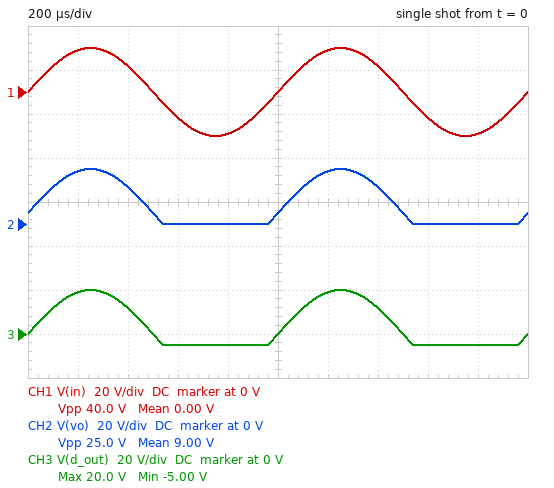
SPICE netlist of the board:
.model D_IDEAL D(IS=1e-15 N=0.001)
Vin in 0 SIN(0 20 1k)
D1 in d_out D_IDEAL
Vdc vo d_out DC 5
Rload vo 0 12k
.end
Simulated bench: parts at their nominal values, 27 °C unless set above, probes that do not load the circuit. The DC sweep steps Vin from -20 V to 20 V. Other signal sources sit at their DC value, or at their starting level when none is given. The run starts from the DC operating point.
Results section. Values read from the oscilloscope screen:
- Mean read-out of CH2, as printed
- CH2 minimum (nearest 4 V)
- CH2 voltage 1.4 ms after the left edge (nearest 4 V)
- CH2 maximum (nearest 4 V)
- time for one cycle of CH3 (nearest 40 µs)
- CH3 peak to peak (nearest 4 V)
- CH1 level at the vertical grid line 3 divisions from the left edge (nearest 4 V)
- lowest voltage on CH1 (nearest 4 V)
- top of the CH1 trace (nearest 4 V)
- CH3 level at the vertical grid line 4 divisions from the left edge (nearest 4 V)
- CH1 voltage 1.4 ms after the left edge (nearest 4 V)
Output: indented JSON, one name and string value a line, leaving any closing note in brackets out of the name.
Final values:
{
  "Mean read-out of CH2, as printed": "9.00 V",
  "CH2 minimum": "0 V",
  "CH2 voltage 1.4 ms after the left edge": "16 V",
  "CH2 maximum": "24 V",
  "time for one cycle of CH3": "1.00 ms",
  "CH3 peak to peak": "24 V",
  "CH1 level at the vertical grid line 3 divisions from the left edge": "-12 V",
  "lowest voltage on CH1": "-20 V",
  "top of the CH1 trace": "20 V",
  "CH3 level at the vertical grid line 4 divisions from the left edge": "-4 V",
  "CH1 voltage 1.4 ms after the left edge": "12 V"
}
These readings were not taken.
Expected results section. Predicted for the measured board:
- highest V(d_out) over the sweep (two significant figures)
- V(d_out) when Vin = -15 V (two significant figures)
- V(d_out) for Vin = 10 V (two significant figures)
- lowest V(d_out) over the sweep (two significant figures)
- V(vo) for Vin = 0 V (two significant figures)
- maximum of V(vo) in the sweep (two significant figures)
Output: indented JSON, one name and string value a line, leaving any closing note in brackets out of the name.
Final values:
{
  "highest V(d_out) over the sweep": "20 V",
  "V(d_out) when Vin = -15 V": "-5.0 V",
  "V(d_out) for Vin = 10 V": "10 V",
  "lowest V(d_out) over the sweep": "-5.0 V",
  "V(vo) for Vin = 0 V": "5.0 V",
  "maximum of V(vo) in the sweep": "25 V"
}
